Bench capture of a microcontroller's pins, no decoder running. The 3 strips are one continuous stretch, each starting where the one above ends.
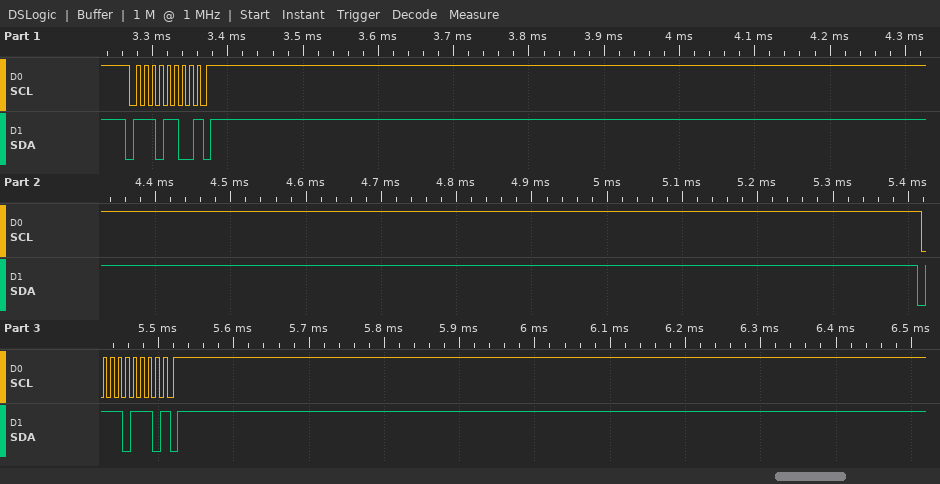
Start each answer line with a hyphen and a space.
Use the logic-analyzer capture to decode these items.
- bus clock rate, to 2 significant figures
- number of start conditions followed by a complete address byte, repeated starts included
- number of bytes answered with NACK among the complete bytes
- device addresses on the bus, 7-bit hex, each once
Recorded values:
- 100 kHz
- 2
- 2
- 0x76 0x77
